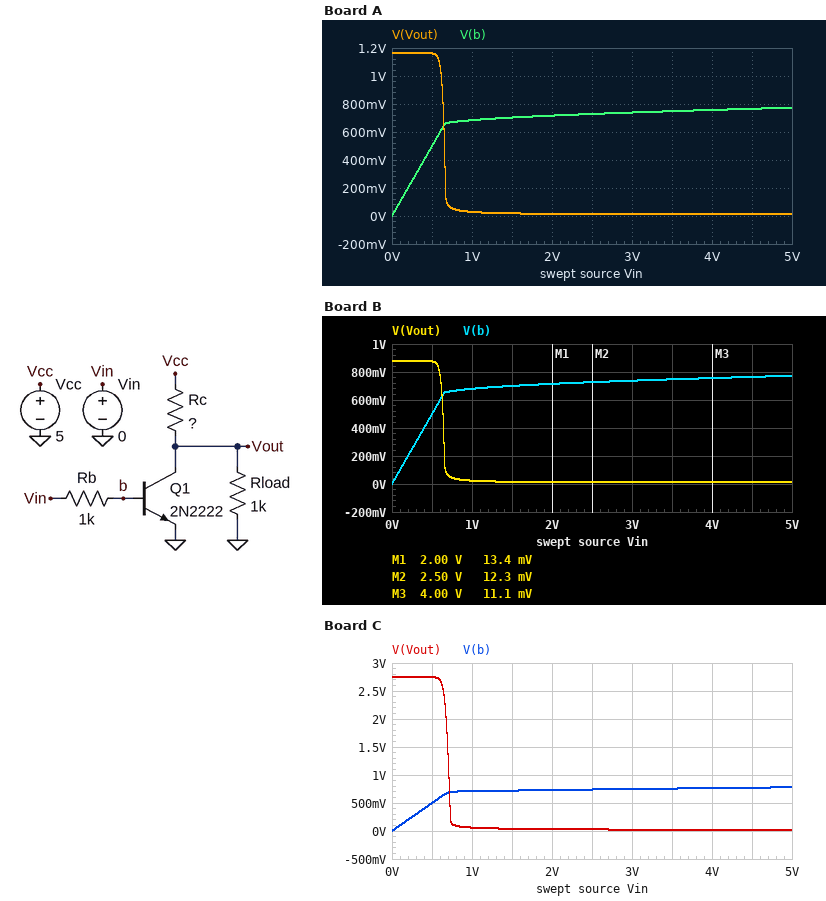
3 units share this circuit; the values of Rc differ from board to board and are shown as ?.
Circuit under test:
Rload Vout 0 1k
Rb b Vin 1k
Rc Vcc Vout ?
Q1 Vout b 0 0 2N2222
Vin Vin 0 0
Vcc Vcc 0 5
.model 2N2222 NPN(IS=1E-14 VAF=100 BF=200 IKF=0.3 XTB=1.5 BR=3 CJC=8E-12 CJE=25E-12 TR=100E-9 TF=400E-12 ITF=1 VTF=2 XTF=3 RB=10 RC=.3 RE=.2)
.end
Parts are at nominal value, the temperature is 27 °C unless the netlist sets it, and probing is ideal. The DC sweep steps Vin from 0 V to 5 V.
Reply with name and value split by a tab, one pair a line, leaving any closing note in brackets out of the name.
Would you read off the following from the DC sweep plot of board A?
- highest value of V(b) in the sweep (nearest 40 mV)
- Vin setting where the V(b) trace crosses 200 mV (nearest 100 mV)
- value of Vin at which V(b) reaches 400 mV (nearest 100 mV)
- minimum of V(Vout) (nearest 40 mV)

highest value of V(b) in the sweep	760 mV
Vin setting where the V(b) trace crosses 200 mV	200 mV
value of Vin at which V(b) reaches 400 mV	400 mV
minimum of V(Vout)	0 V
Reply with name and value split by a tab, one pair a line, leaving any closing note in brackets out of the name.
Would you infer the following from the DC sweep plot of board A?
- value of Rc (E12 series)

value of Rc	3.3 kΩ
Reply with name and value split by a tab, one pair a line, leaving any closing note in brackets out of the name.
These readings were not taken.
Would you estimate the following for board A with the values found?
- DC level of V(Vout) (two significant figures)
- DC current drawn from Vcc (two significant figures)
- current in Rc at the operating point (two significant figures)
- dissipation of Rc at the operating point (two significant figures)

DC level of V(Vout)	1.2 V
DC current drawn from Vcc	1.2 mA
current in Rc at the operating point	1.2 mA
dissipation of Rc at the operating point	4.5 mW
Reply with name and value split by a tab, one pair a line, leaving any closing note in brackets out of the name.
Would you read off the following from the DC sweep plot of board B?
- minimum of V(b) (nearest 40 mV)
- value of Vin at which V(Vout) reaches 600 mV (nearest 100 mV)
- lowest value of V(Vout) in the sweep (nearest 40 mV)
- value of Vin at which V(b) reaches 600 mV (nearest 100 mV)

minimum of V(b)	0 V
value of Vin at which V(Vout) reaches 600 mV	600 mV
lowest value of V(Vout) in the sweep	0 V
value of Vin at which V(b) reaches 600 mV	600 mV
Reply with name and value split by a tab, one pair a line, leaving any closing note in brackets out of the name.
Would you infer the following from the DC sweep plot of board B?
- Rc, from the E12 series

Rc, from the E12 series	4.7 kΩ
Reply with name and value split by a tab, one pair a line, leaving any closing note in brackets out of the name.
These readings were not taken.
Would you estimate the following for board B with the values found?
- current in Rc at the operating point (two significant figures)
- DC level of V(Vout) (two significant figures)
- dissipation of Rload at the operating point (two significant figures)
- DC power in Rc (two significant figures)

current in Rc at the operating point	880 µA
DC level of V(Vout)	880 mV
dissipation of Rload at the operating point	770 µW
DC power in Rc	3.6 mW
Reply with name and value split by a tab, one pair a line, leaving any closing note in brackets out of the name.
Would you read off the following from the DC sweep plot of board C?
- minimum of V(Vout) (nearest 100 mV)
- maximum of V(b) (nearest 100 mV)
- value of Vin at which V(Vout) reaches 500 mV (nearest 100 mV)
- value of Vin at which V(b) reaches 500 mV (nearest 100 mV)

minimum of V(Vout)	0 V
maximum of V(b)	800 mV
value of Vin at which V(Vout) reaches 500 mV	700 mV
value of Vin at which V(b) reaches 500 mV	500 mV
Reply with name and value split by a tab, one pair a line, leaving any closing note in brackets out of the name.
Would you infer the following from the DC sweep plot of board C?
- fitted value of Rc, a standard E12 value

fitted value of Rc, a standard E12 value	820 Ω
